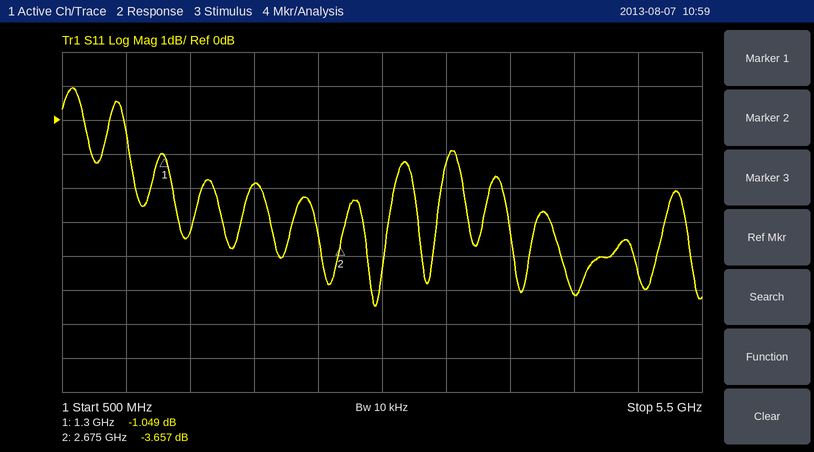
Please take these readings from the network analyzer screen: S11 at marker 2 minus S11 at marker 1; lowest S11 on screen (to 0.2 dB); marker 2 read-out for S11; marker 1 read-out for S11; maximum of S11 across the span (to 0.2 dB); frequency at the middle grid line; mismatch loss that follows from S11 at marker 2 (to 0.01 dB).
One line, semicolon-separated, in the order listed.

-2.608 dB; -5.4 dB; -3.657 dB; -1.049 dB; 1.0 dB; 3 GHz; 2.45 dB
